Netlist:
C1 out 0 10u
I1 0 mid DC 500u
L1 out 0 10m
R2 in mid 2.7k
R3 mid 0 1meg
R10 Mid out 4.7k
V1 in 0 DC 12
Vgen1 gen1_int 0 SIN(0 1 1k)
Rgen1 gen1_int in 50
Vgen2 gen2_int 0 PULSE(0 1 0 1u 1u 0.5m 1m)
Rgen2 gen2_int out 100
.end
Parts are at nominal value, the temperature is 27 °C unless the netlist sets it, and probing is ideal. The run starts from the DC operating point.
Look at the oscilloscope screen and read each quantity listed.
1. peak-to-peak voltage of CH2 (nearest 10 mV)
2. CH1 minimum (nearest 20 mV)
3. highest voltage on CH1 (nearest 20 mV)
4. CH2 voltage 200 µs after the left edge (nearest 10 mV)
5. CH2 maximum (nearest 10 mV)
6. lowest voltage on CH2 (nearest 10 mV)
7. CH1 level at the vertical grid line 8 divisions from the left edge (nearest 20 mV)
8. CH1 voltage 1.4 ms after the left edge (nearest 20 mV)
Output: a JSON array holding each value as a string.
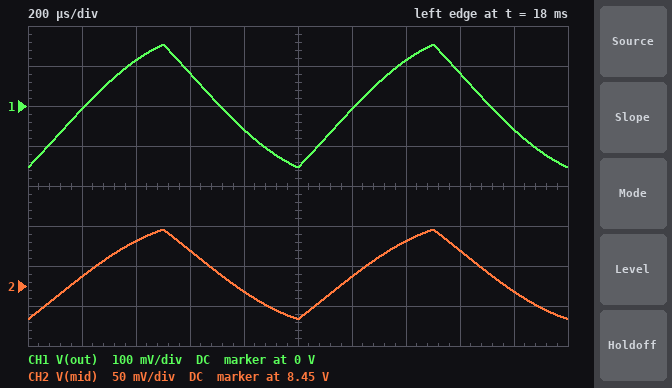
["110 mV", "-160 mV", "160 mV", "8.46 V", "8.52 V", "8.41 V", "80 mV", "120 mV"]
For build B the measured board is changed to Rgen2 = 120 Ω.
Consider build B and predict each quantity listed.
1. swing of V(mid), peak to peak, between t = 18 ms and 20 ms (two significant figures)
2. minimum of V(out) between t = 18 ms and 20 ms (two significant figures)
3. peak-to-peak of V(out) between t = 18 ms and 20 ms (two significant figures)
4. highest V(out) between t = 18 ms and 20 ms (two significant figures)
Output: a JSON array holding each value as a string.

["94 mV", "-130 mV", "260 mV", "130 mV"]
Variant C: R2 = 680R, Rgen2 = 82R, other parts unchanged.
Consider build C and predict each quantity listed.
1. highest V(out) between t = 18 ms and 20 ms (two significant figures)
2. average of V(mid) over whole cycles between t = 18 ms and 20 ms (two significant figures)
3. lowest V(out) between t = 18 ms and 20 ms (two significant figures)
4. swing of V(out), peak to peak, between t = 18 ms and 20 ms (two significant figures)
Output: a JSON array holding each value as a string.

["180 mV", "11 V", "-180 mV", "370 mV"]
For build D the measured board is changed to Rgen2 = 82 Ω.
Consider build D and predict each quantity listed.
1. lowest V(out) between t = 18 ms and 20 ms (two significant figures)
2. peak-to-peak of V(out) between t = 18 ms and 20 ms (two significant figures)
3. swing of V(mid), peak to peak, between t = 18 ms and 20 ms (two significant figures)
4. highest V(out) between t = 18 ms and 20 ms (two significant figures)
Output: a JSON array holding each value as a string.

["-180 mV", "370 mV", "130 mV", "180 mV"]
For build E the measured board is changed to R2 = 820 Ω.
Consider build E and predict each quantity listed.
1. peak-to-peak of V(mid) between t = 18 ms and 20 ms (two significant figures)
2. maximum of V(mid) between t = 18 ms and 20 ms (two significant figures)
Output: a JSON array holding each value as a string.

["46 mV", "11 V"]
